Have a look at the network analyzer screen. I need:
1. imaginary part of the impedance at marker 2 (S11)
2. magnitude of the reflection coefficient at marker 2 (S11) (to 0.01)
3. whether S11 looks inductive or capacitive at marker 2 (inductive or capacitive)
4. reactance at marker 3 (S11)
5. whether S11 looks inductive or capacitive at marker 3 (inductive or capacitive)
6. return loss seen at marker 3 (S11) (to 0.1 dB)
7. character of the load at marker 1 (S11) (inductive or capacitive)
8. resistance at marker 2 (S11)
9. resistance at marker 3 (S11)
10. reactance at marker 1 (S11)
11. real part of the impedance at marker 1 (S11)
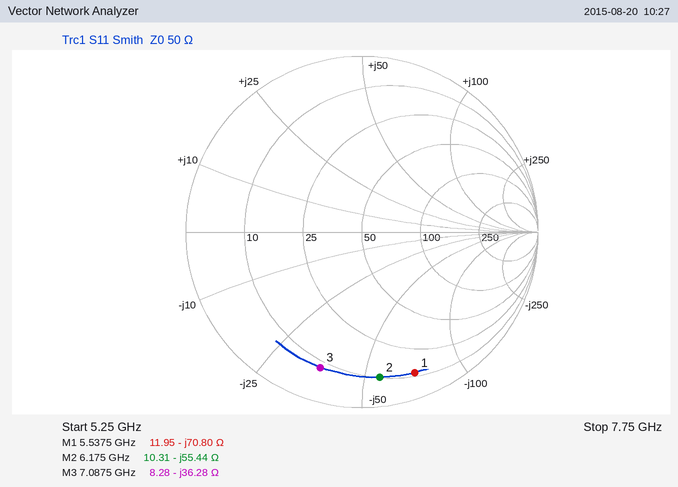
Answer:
-55.44 Ω
0.83
capacitive
-36.28 Ω
capacitive
1.9 dB
capacitive
10.31 Ω
8.28 Ω
-70.80 Ω
11.95 Ω
